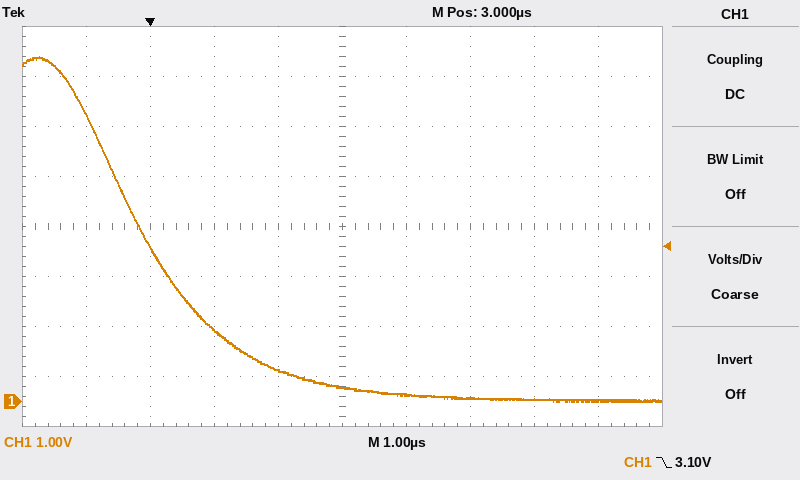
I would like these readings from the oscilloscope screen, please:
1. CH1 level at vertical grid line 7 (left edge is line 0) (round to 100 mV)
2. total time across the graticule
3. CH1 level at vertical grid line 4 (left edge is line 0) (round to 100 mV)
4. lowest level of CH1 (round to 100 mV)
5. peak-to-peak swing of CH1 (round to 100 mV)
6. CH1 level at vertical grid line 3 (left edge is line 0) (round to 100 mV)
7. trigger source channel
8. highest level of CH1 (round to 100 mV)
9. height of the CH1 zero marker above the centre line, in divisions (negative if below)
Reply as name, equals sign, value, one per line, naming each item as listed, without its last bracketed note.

CH1 level at vertical grid line 7 (left edge is line 0) = 100 mV
total time across the graticule = 10 µs
CH1 level at vertical grid line 4 (left edge is line 0) = 600 mV
lowest level of CH1 = 0.0 V
peak-to-peak swing of CH1 = 6.9 V
CH1 level at vertical grid line 3 (left edge is line 0) = 1.4 V
trigger source channel = CH1
highest level of CH1 = 6.9 V
height of the CH1 zero marker above the centre line, in divisions = -3.5 div
